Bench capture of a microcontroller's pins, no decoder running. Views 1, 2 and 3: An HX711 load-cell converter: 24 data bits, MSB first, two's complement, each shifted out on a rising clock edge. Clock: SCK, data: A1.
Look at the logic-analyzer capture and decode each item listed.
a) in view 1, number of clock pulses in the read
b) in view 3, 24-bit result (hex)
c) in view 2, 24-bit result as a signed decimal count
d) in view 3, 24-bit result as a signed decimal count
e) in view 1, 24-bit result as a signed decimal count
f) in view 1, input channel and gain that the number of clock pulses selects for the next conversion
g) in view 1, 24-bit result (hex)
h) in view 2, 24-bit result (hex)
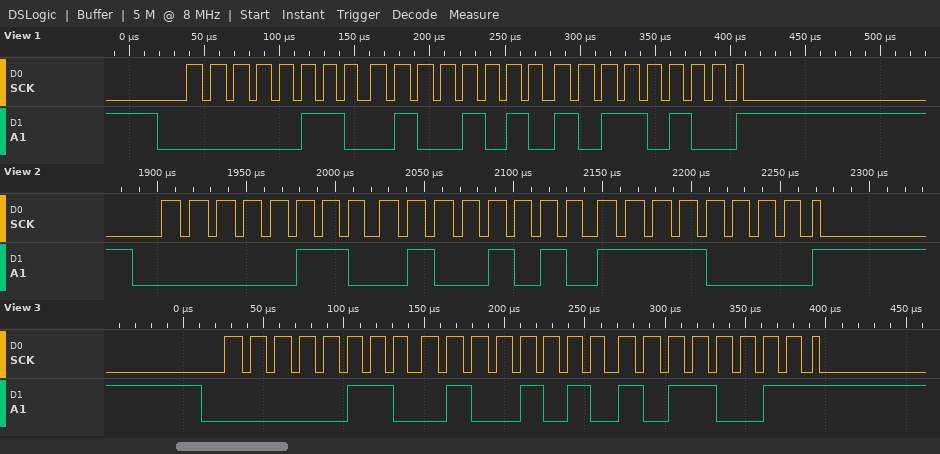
25
0x064AB3
412400
412339
412340
channel A, gain 128
0x064AB4
0x064AF0
